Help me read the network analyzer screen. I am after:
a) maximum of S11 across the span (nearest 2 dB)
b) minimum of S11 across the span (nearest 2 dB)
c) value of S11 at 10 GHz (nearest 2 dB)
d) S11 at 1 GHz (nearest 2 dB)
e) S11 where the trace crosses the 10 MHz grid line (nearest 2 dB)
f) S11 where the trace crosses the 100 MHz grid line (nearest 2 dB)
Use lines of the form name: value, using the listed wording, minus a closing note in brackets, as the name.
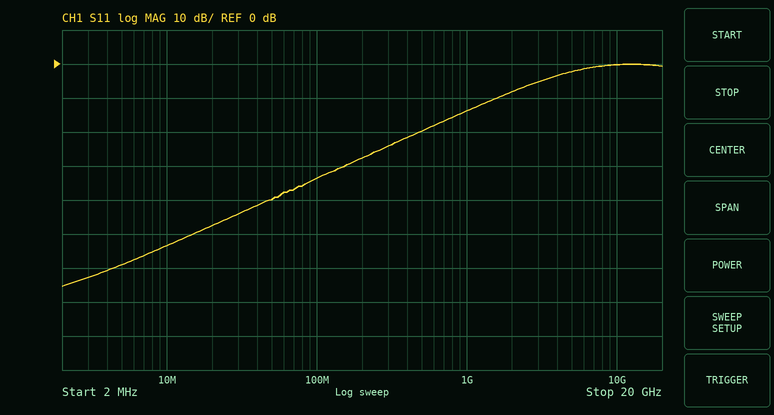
maximum of S11 across the span: 0 dB
minimum of S11 across the span: -66 dB
value of S11 at 10 GHz: 0 dB
S11 at 1 GHz: -14 dB
S11 where the trace crosses the 10 MHz grid line: -54 dB
S11 where the trace crosses the 100 MHz grid line: -34 dB
